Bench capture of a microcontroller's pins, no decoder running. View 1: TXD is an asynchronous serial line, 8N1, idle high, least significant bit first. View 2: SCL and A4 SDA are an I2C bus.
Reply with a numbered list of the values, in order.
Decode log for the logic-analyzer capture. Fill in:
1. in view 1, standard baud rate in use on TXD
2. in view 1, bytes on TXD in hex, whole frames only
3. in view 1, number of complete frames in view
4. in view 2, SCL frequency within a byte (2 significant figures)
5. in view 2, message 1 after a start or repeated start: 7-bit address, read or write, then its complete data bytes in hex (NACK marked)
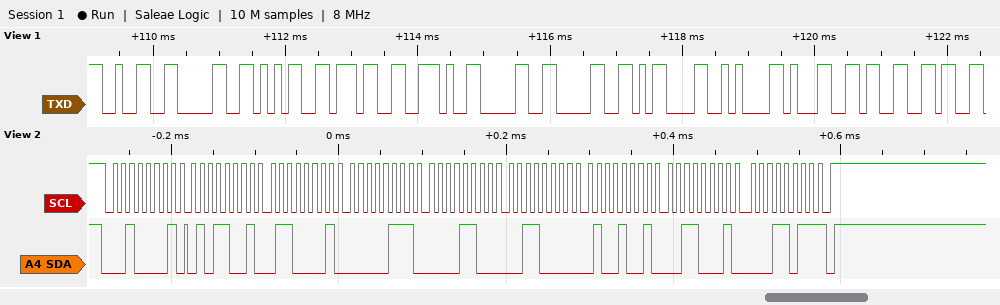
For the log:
1. 9600 baud
2. 0x32 0x30 0x35 0x37 0x2E 0x30 0x30 0x0D 0x0A 0x31 0x33
3. 11
4. 100 kHz
5. 0x10 read: 59 61 07 0C 30 49 31 1B NACK
